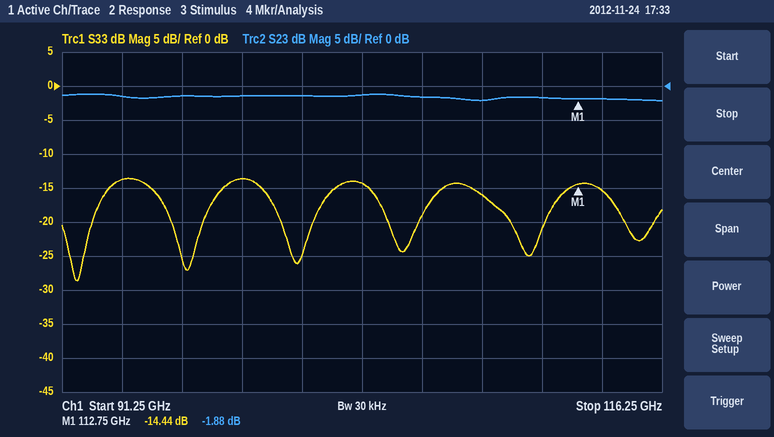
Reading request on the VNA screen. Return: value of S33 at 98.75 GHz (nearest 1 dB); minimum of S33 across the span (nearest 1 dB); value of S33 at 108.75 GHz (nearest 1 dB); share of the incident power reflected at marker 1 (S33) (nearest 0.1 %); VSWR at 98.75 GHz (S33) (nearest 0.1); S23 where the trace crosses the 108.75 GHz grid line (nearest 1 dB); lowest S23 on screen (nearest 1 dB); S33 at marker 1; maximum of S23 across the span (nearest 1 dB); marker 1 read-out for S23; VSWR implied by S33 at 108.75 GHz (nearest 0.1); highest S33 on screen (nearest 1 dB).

-14 dB
-29 dB
-16 dB
3.6 %
1.5
-2 dB
-2 dB
-14.44 dB
-1 dB
-1.88 dB
1.4
-14 dB
